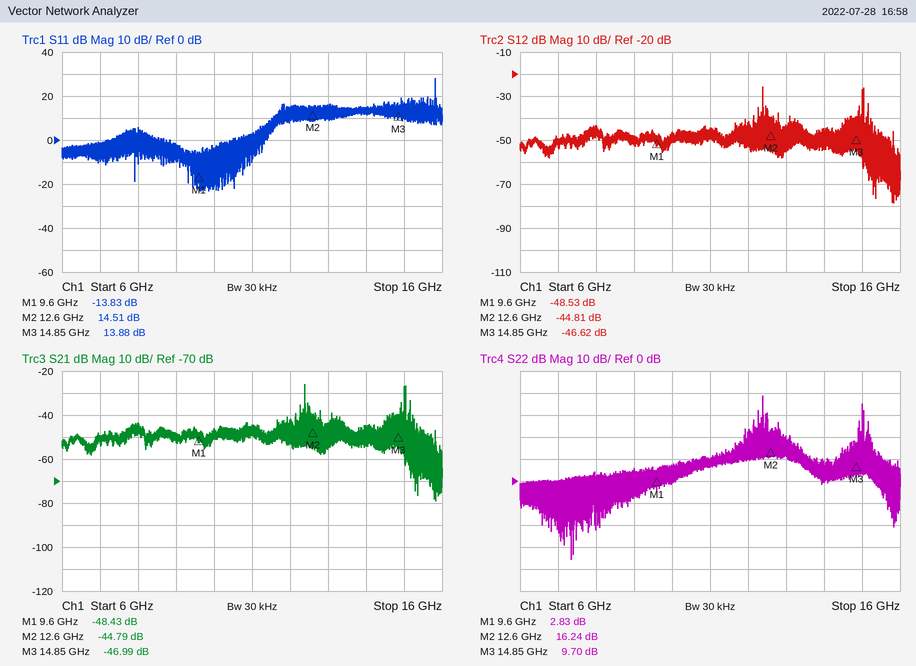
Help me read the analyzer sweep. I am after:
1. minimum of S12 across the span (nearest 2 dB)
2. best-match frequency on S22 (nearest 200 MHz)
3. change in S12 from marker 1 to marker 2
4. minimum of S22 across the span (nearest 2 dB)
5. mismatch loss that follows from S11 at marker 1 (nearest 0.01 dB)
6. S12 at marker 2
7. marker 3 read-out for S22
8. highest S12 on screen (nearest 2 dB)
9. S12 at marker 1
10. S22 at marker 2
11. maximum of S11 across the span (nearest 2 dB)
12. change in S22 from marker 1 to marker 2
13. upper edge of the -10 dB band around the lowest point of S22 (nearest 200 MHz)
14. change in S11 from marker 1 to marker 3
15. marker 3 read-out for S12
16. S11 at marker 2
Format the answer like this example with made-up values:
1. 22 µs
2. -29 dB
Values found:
1. -78 dB
2. 7.4 GHz
3. 3.72 dB
4. -36 dB
5. 0.18 dB
6. -44.81 dB
7. 9.70 dB
8. -26 dB
9. -48.53 dB
10. 16.24 dB
11. 28 dB
12. 13.41 dB
13. 7.4 GHz
14. 27.71 dB
15. -46.62 dB
16. 14.51 dB
